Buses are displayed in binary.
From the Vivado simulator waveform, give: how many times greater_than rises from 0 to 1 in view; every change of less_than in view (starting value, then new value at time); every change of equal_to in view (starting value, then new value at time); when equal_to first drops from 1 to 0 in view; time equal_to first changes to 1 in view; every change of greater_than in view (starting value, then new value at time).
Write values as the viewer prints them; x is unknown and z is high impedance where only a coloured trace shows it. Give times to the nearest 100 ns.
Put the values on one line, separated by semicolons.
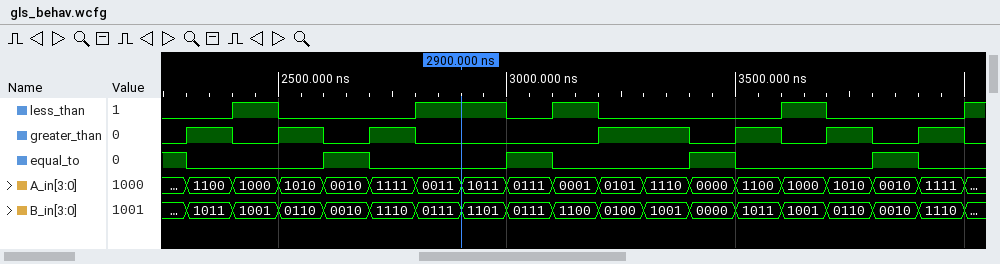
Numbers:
7; 0, 1 at 2400 ns, 0 at 2500 ns, 1 at 2800 ns, 0 at 3000 ns, 1 at 3100 ns, 0 at 3200 ns, 1 at 3600 ns, 0 at 3700 ns, 1 at 4000 ns; 1, 0 at 2300 ns, 1 at 2600 ns, 0 at 2700 ns, 1 at 3000 ns, 0 at 3100 ns, 1 at 3400 ns, 0 at 3500 ns, 1 at 3800 ns, 0 at 3900 ns; 2300 ns; 2600 ns; 0, 1 at 2300 ns, 0 at 2400 ns, 1 at 2500 ns, 0 at 2600 ns, 1 at 2700 ns, 0 at 2800 ns, 1 at 3200 ns, 0 at 3400 ns, 1 at 3500 ns, 0 at 3600 ns, 1 at 3700 ns, 0 at 3800 ns, 1 at 3900 ns, 0 at 4000 ns
